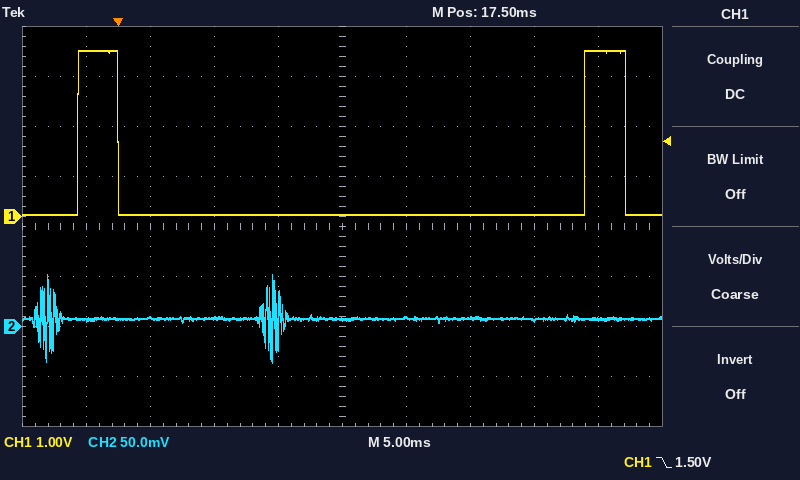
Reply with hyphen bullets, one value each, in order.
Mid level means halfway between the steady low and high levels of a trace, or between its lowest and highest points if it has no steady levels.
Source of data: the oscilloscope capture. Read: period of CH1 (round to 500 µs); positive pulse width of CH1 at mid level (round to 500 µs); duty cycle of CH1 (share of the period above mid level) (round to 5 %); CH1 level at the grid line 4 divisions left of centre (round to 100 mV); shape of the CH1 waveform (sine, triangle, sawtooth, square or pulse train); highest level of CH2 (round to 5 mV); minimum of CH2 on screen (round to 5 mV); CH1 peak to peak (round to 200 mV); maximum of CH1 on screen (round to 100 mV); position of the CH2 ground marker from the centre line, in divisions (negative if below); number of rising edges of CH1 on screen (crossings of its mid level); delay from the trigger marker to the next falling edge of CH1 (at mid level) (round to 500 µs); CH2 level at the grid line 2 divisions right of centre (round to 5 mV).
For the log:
- 39.5 ms
- 3.0 ms
- 10 %
- 3.3 V
- pulse train
- 50 mV
- -35 mV
- 3.2 V
- 3.3 V
- -2.0 div
- 2
- 39.5 ms
- 10 mV
